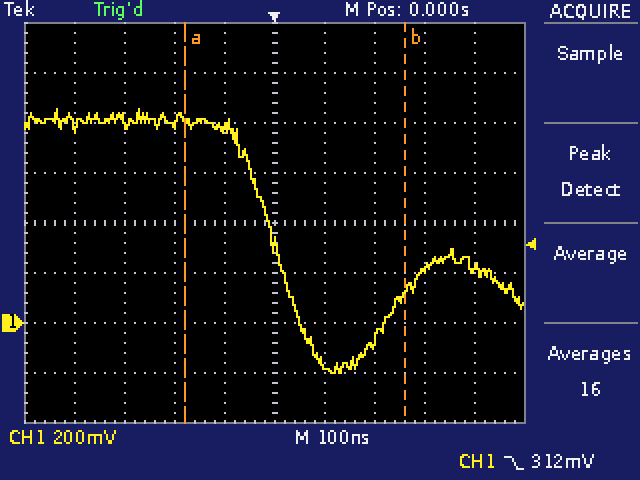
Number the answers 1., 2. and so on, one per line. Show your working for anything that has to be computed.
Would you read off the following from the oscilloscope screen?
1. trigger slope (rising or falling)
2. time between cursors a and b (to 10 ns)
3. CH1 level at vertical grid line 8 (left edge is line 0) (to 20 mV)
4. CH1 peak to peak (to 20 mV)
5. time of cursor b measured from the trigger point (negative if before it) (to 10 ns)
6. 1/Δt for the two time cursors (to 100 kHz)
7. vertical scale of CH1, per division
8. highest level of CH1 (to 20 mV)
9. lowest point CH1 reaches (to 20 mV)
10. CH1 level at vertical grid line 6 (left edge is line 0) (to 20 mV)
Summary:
1. falling
2. 440 ns
3. 220 mV
4. 860 mV − (-200 mV) = 1.06 V
5. +260 ns
6. 1 / 440 ns ≈ 2.3 MHz
7. 200 mV
8. 860 mV
9. -200 mV
10. -160 mV
